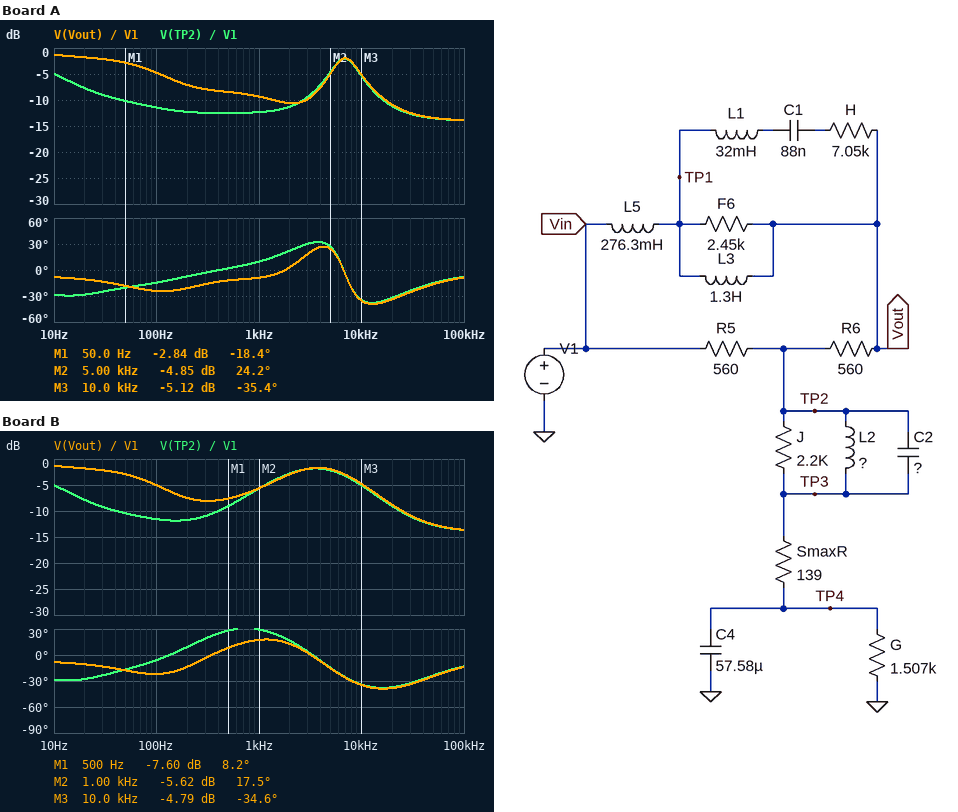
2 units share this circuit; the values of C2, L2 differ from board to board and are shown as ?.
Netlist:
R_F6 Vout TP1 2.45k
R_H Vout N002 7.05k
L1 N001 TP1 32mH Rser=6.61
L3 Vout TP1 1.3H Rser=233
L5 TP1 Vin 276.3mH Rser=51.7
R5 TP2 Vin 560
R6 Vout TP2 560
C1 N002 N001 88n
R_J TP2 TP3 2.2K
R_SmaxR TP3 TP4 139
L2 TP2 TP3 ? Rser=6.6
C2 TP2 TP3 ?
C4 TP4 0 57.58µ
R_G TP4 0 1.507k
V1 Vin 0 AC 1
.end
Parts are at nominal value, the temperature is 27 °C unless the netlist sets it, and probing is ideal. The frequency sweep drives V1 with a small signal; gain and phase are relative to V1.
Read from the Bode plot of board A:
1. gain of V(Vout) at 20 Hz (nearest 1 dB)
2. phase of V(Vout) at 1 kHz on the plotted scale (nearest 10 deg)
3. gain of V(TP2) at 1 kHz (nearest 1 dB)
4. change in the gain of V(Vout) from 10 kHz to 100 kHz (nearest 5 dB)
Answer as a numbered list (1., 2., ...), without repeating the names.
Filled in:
1. -2 dB
2. -10 deg
3. -12 dB
4. -10 dB
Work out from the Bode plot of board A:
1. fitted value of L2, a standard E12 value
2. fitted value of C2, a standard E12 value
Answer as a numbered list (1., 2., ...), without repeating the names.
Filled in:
1. 8.2 mH
2. 68 nF
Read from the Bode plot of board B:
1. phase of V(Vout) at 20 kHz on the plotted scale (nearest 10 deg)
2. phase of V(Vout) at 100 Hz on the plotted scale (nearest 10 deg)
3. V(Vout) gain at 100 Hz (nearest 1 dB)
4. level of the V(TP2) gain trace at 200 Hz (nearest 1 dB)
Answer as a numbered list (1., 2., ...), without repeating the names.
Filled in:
1. -40 deg
2. -20 deg
3. -5 dB
4. -12 dB
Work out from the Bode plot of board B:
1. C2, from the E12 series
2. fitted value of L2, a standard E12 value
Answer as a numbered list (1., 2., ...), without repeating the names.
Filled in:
1. 39 nF
2. 56 mH
